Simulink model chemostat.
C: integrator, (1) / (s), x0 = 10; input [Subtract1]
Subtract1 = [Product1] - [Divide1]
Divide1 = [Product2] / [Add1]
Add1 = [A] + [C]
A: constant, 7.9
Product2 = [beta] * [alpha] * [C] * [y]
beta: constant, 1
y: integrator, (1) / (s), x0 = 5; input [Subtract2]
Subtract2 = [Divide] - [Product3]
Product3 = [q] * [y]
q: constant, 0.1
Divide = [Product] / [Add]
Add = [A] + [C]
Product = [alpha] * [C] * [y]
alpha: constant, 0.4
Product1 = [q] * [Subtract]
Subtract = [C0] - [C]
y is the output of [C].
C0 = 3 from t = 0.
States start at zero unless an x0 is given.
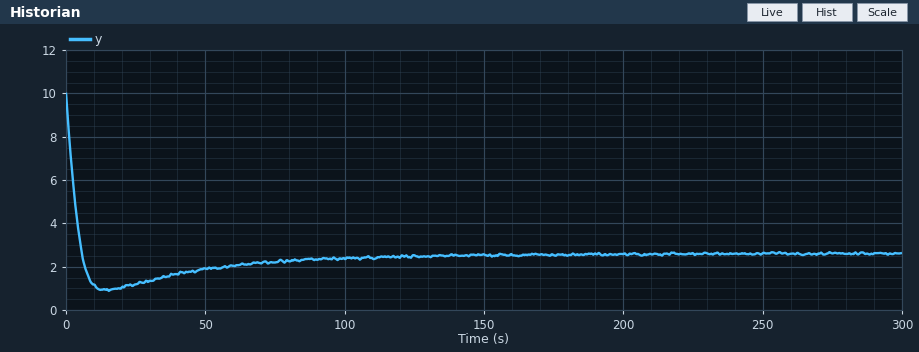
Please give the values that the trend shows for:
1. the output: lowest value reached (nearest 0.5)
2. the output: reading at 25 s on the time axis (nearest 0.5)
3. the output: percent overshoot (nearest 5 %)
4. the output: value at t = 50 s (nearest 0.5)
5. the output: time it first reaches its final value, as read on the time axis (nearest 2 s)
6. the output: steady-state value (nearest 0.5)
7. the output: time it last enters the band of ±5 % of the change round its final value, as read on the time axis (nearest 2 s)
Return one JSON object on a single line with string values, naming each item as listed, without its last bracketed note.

{"the output: lowest value reached": "1.0", "the output: reading at 25 s on the time axis": "1.0", "the output: percent overshoot": "25 %", "the output: value at t = 50 s": "2.0", "the output: time it first reaches its final value, as read on the time axis": "6 s", "the output: steady-state value": "2.5", "the output: time it last enters the band of ±5 % of the change round its final value, as read on the time axis": "80 s"}
